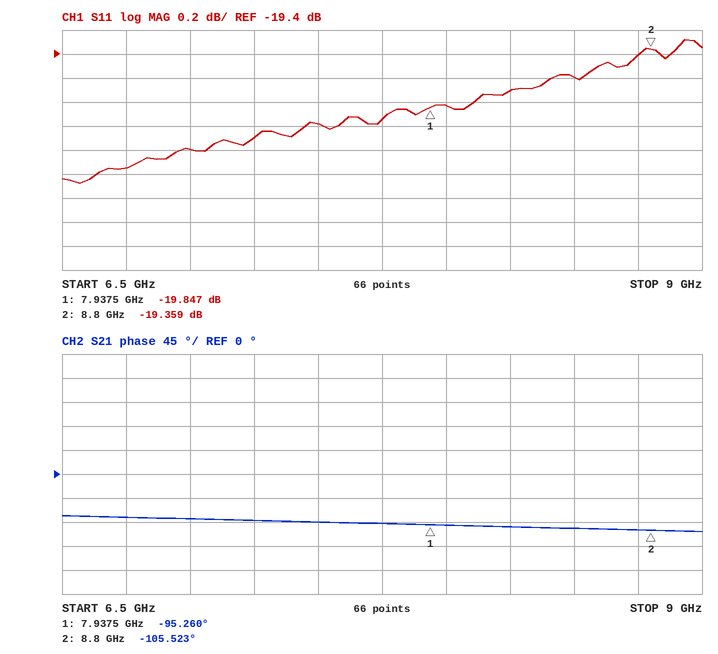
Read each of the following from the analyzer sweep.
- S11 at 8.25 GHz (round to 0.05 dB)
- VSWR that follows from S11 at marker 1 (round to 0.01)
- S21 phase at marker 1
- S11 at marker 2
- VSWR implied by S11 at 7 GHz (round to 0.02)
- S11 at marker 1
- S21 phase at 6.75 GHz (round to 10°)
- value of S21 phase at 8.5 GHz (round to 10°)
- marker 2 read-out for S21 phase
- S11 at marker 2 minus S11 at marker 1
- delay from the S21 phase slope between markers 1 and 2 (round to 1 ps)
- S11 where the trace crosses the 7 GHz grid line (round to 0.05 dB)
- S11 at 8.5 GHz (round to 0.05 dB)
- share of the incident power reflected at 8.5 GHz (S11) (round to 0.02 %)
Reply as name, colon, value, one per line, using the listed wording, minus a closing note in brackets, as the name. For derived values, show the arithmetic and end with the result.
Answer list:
S11 at 8.25 GHz: -19.70 dB
VSWR that follows from S11 at marker 1: (1 + 0.1018)/(1 − 0.1018) ≈ 1.23
S21 phase at marker 1: -95.260°
S11 at marker 2: -19.359 dB
VSWR implied by S11 at 7 GHz: |Γ| = 10^(-20.2/20) = 0.0977; VSWR = (1 + 0.0977)/(1 − 0.0977) ≈ 1.22
S11 at marker 1: -19.847 dB
S21 phase at 6.75 GHz: -80°
value of S21 phase at 8.5 GHz: -100°
marker 2 read-out for S21 phase: -105.523°
S11 at marker 2 minus S11 at marker 1: -19.359 − (-19.847) = 0.488 dB
delay from the S21 phase slope between markers 1 and 2: −(-105.523° − (-95.26°))/(360° × 862.5 MHz) ≈ 33 ps
S11 where the trace crosses the 7 GHz grid line: -20.20 dB
S11 at 8.5 GHz: -19.60 dB
share of the incident power reflected at 8.5 GHz (S11): 10^(-19.6/10) ≈ 1.10 %
